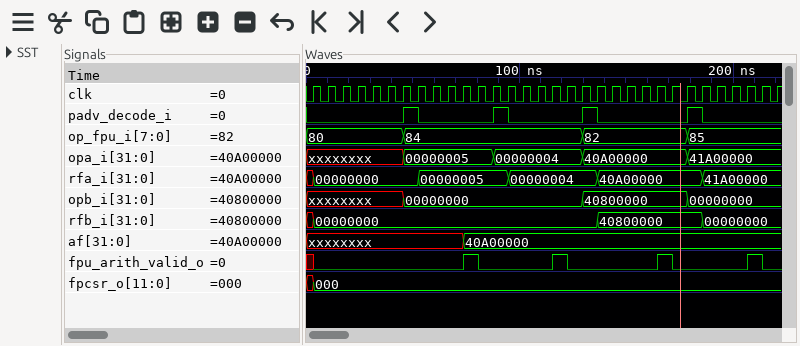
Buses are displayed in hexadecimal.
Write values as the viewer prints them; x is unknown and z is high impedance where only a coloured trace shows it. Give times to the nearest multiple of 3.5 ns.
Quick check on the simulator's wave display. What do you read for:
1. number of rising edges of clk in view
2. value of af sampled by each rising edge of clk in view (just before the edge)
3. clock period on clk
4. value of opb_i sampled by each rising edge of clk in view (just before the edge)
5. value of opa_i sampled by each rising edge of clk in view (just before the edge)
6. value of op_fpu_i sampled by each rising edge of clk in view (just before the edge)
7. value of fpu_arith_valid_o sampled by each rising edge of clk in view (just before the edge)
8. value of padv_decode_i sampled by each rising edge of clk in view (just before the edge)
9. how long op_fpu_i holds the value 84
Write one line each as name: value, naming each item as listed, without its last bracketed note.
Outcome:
number of rising edges of clk in view: 32
value of af sampled by each rising edge of clk in view: xxxxxxxx, xxxxxxxx, xxxxxxxx, xxxxxxxx, xxxxxxxx, xxxxxxxx, xxxxxxxx, xxxxxxxx, xxxxxxxx, xxxxxxxx, xxxxxxxx, 40A00000, 40A00000, 40A00000, 40A00000, 40A00000, 40A00000, 40A00000, 40A00000, 40A00000, 40A00000, 40A00000, 40A00000, 40A00000, 40A00000, 40A00000, 40A00000, 40A00000, 40A00000, 40A00000, 40A00000, 40A00000
clock period on clk: 7 ns
value of opb_i sampled by each rising edge of clk in view: xxxxxxxx, xxxxxxxx, xxxxxxxx, xxxxxxxx, xxxxxxxx, xxxxxxxx, xxxxxxxx, 00000000, 00000000, 00000000, 00000000, 00000000, 00000000, 00000000, 00000000, 00000000, 00000000, 00000000, 00000000, 40800000, 40800000, 40800000, 40800000, 40800000, 40800000, 40800000, 00000000, 00000000, 00000000, 00000000, 00000000, 00000000
value of opa_i sampled by each rising edge of clk in view: xxxxxxxx, xxxxxxxx, xxxxxxxx, xxxxxxxx, xxxxxxxx, xxxxxxxx, xxxxxxxx, 00000005, 00000005, 00000005, 00000005, 00000005, 00000005, 00000004, 00000004, 00000004, 00000004, 00000004, 00000004, 40A00000, 40A00000, 40A00000, 40A00000, 40A00000, 40A00000, 40A00000, 41A00000, 41A00000, 41A00000, 41A00000, 41A00000, 41A00000
value of op_fpu_i sampled by each rising edge of clk in view: 80, 80, 80, 80, 80, 80, 80, 84, 84, 84, 84, 84, 84, 84, 84, 84, 84, 84, 84, 82, 82, 82, 82, 82, 82, 82, 85, 85, 85, 85, 85, 85
value of fpu_arith_valid_o sampled by each rising edge of clk in view: x 0 0 0 0 0 0 0 0 0 0 1 0 0 0 0 0 1 0 0 0 0 0 0 1 0 0 0 0 0 1 0
value of padv_decode_i sampled by each rising edge of clk in view: 0 0 0 0 0 0 0 1 0 0 0 0 0 1 0 0 0 0 0 1 0 0 0 0 0 0 1 0 0 0 0 0
how long op_fpu_i holds the value 84: 84 ns
